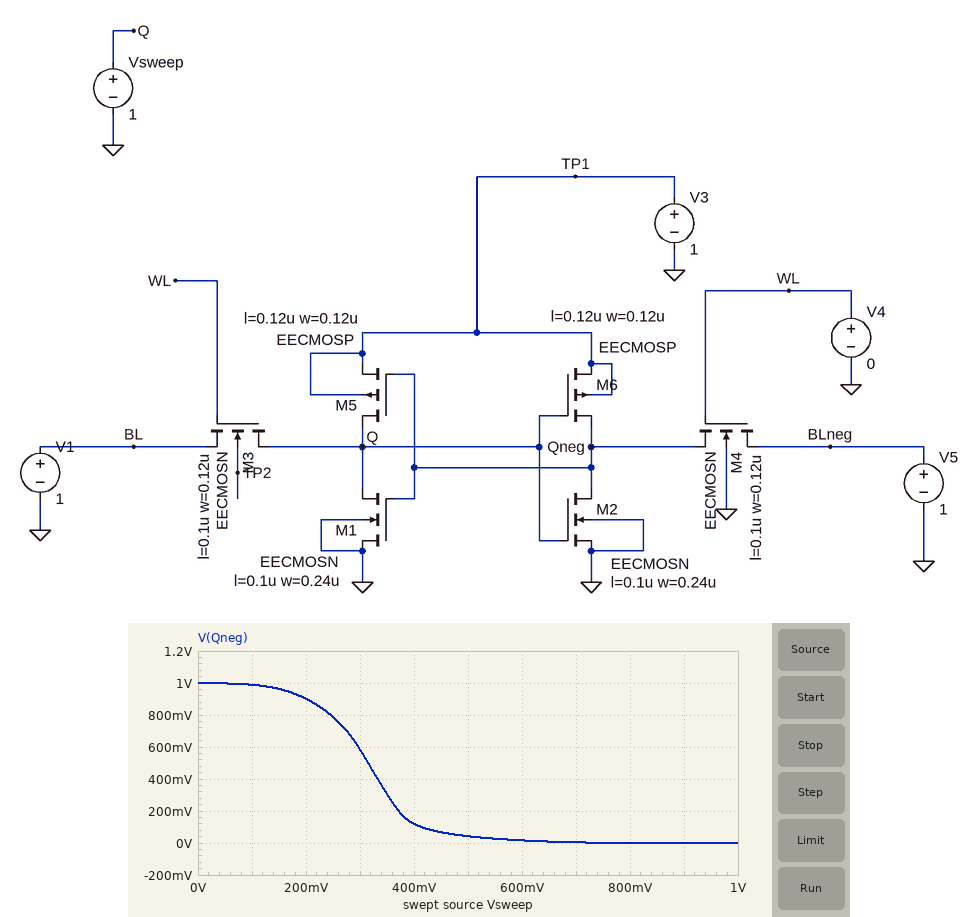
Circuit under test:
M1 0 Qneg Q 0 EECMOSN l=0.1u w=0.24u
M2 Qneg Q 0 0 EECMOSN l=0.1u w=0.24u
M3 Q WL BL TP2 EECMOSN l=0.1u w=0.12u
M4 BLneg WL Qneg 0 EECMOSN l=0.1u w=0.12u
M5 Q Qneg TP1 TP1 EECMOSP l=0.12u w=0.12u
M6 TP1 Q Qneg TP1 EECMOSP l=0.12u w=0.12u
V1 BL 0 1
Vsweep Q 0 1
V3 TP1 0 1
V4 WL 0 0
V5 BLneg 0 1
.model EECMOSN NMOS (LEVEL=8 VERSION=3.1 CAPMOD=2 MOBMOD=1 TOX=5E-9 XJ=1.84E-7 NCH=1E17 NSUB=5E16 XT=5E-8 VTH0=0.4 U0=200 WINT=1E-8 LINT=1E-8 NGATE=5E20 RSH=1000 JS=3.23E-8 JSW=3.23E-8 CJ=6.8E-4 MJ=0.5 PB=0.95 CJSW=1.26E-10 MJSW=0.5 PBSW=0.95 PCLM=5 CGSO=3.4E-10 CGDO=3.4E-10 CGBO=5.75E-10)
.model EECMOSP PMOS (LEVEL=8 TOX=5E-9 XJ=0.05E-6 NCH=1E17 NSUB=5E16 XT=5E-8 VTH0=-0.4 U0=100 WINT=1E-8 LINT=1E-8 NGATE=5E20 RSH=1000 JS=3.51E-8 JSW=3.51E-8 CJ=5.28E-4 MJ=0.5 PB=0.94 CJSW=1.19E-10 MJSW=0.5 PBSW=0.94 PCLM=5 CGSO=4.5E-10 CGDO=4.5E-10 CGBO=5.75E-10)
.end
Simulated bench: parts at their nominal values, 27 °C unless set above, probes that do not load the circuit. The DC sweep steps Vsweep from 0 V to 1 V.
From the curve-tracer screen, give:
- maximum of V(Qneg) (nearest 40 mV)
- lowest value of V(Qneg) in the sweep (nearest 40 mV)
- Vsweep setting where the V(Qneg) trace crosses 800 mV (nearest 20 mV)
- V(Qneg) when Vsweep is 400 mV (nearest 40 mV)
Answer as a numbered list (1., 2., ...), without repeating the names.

1. 1.00 V
2. 0 V
3. 240 mV
4. 120 mV
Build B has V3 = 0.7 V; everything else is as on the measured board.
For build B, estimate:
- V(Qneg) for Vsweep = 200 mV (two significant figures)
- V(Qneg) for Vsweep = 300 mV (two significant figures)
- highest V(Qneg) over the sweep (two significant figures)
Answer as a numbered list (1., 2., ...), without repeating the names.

1. 590 mV
2. 57 mV
3. 700 mV
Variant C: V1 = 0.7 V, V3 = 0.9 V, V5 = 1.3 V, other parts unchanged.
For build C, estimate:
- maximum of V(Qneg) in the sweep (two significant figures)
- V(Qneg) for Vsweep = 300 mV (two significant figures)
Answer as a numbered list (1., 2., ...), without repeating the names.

1. 900 mV
2. 410 mV
